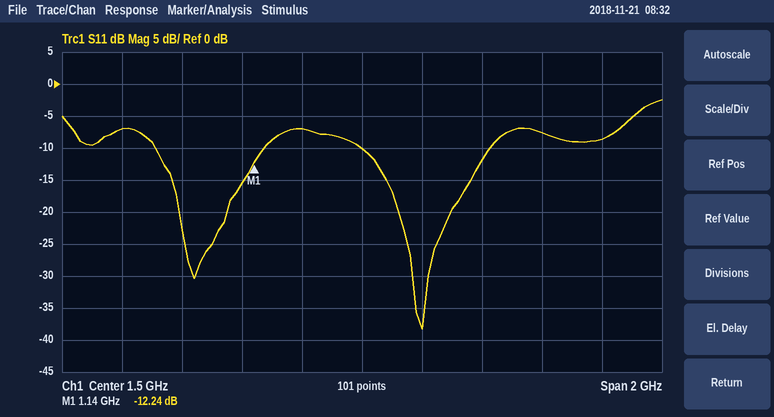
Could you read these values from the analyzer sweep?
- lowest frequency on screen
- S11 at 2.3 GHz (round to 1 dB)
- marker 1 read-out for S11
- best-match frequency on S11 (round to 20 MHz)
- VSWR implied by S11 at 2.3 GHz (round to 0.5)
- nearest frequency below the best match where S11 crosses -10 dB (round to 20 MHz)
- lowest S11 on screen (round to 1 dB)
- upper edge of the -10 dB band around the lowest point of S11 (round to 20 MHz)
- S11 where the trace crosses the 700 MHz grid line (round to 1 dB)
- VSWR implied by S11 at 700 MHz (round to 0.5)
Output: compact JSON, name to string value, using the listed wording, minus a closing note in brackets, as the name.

{"lowest frequency on screen": "500 MHz", "S11 at 2.3 GHz": "-9 dB", "marker 1 read-out for S11": "-12.24 dB", "best-match frequency on S11": "1.70 GHz", "VSWR implied by S11 at 2.3 GHz": "2.0", "nearest frequency below the best match where S11 crosses -10 dB": "1.50 GHz", "lowest S11 on screen": "-38 dB", "upper edge of the -10 dB band around the lowest point of S11": "1.92 GHz", "S11 where the trace crosses the 700 MHz grid line": "-7 dB", "VSWR implied by S11 at 700 MHz": "2.5"}
